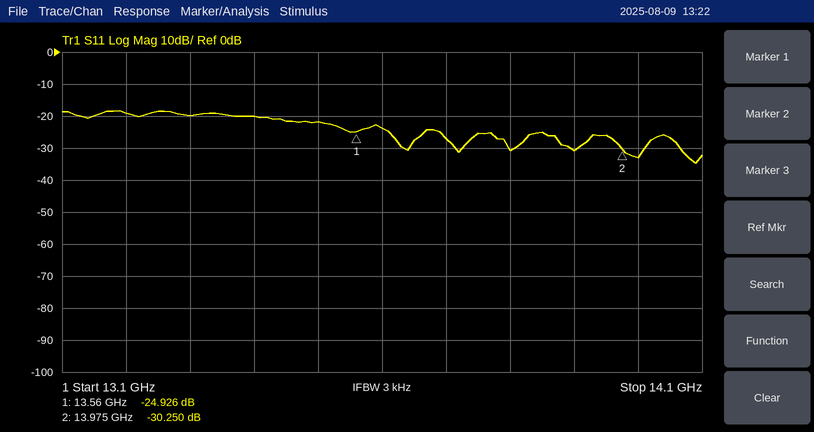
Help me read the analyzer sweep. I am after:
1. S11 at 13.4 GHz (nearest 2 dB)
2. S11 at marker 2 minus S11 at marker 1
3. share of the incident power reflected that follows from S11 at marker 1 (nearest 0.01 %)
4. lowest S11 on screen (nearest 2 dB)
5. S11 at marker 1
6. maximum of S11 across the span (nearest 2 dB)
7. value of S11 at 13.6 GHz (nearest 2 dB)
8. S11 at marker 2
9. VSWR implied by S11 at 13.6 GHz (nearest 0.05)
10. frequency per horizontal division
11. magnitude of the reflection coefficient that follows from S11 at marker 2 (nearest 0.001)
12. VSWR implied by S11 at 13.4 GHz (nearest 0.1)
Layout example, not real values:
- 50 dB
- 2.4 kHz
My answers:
- -20 dB
- -5.324 dB
- 0.32 %
- -34 dB
- -24.926 dB
- -18 dB
- -24 dB
- -30.250 dB
- 1.15
- 100 MHz
- 0.031
- 1.2
